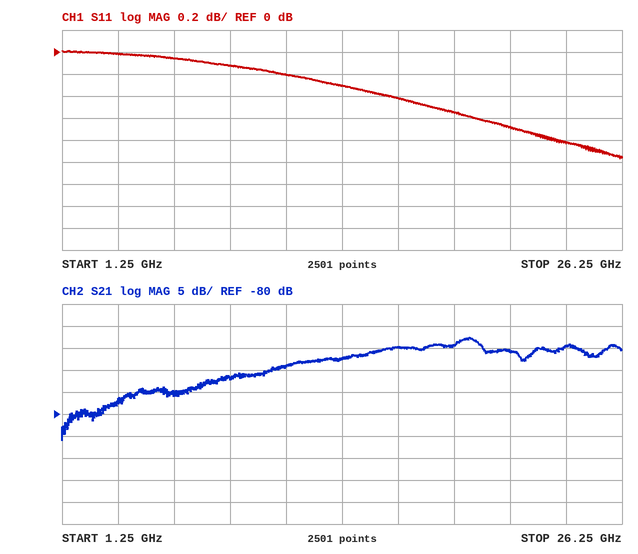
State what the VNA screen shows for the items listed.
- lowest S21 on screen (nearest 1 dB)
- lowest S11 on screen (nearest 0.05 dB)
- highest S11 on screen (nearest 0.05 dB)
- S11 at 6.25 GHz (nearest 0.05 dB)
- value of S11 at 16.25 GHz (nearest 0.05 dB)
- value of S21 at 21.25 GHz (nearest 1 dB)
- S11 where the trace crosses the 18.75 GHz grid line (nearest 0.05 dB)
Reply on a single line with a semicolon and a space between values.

-86 dB; -0.95 dB; 0.00 dB; -0.05 dB; -0.40 dB; -66 dB; -0.55 dB
